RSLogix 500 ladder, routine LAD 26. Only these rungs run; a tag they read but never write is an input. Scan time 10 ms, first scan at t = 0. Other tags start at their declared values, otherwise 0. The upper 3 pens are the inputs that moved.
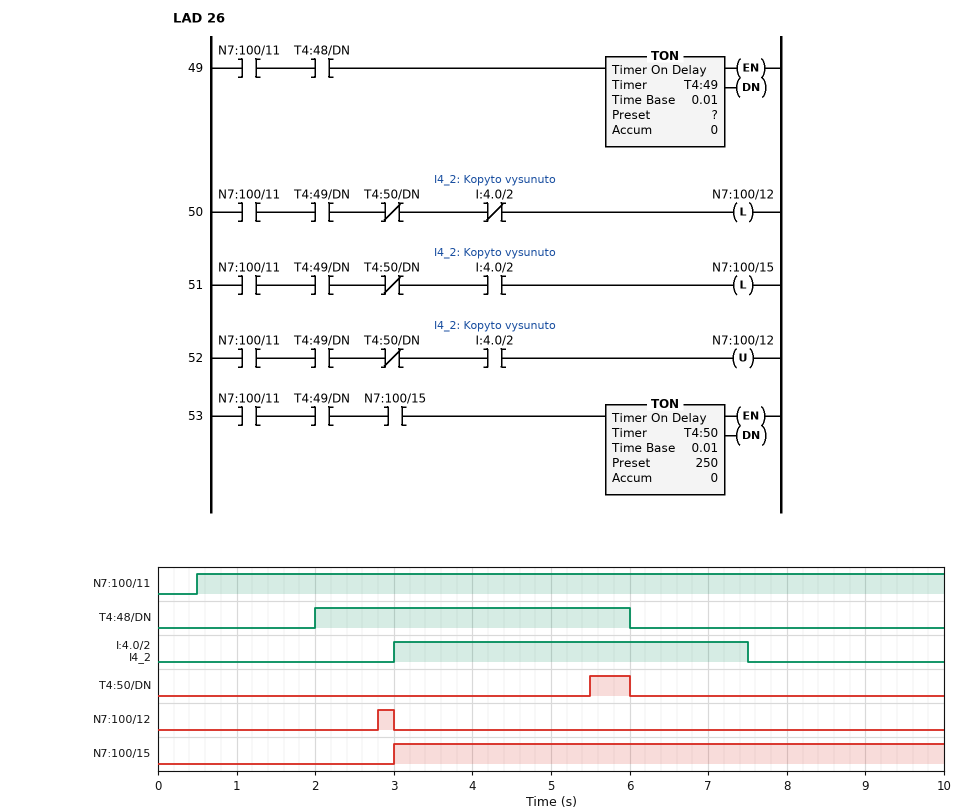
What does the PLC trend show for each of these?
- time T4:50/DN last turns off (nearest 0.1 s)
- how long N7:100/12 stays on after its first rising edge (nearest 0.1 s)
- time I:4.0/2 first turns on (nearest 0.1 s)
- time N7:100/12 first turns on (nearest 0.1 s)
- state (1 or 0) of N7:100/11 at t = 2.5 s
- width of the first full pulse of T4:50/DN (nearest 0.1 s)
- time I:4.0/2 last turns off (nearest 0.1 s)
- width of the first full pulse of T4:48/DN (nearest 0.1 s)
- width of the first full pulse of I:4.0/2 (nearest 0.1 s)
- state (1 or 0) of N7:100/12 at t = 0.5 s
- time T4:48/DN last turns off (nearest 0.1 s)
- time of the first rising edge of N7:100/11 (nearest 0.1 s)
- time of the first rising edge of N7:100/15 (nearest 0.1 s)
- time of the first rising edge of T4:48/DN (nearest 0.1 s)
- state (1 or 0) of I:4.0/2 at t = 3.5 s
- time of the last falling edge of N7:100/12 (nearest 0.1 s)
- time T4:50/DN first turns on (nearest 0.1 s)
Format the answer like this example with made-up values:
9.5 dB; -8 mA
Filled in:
6.0 s; 0.2 s; 3.0 s; 2.8 s; 1; 0.5 s; 7.5 s; 4.0 s; 4.5 s; 0; 6.0 s; 0.5 s; 3.0 s; 2.0 s; 1; 3.0 s; 5.5 s
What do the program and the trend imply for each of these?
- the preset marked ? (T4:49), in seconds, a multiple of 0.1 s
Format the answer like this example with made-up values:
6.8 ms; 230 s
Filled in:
0.8 s
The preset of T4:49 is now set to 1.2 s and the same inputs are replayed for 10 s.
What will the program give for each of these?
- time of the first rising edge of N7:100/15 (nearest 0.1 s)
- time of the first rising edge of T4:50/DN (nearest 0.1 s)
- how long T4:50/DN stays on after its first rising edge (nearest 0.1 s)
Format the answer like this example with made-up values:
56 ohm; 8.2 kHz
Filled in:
3.2 s; 5.7 s; 0.3 s
